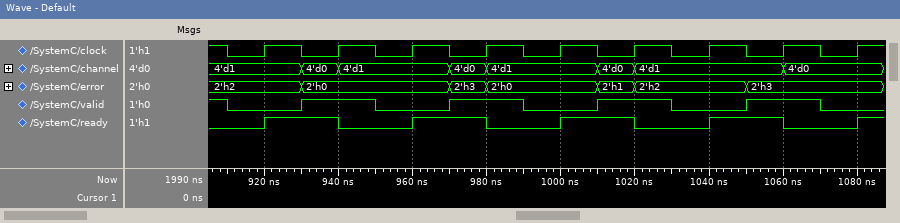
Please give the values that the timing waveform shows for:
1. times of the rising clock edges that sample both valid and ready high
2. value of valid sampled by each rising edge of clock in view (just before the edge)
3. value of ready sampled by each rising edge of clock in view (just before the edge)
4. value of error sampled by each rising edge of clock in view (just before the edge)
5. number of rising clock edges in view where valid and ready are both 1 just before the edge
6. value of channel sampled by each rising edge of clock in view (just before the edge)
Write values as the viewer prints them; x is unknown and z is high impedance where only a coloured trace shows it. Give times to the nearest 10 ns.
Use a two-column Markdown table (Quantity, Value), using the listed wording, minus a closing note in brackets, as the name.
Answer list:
| Quantity | Value |
|---|---|
| times of the rising clock edges that sample both valid and ready high | 940 ns, 980 ns, 1020 ns, 1060 ns |
| value of valid sampled by each rising edge of clock in view | 0 1 0 1 0 1 0 1 0 |
| value of ready sampled by each rising edge of clock in view | 0 1 0 1 0 1 0 1 0 |
| value of error sampled by each rising edge of clock in view | 2'h2, 2'h0, 2'h0, 2'h3, 2'h0, 2'h1, 2'h2, 2'h3, 2'h3 |
| number of rising clock edges in view where valid and ready are both 1 just before the edge | 4 |
| value of channel sampled by each rising edge of clock in view | 4'd1, 4'd0, 4'd1, 4'd0, 4'd1, 4'd0, 4'd1, 4'd1, 4'd0 |
